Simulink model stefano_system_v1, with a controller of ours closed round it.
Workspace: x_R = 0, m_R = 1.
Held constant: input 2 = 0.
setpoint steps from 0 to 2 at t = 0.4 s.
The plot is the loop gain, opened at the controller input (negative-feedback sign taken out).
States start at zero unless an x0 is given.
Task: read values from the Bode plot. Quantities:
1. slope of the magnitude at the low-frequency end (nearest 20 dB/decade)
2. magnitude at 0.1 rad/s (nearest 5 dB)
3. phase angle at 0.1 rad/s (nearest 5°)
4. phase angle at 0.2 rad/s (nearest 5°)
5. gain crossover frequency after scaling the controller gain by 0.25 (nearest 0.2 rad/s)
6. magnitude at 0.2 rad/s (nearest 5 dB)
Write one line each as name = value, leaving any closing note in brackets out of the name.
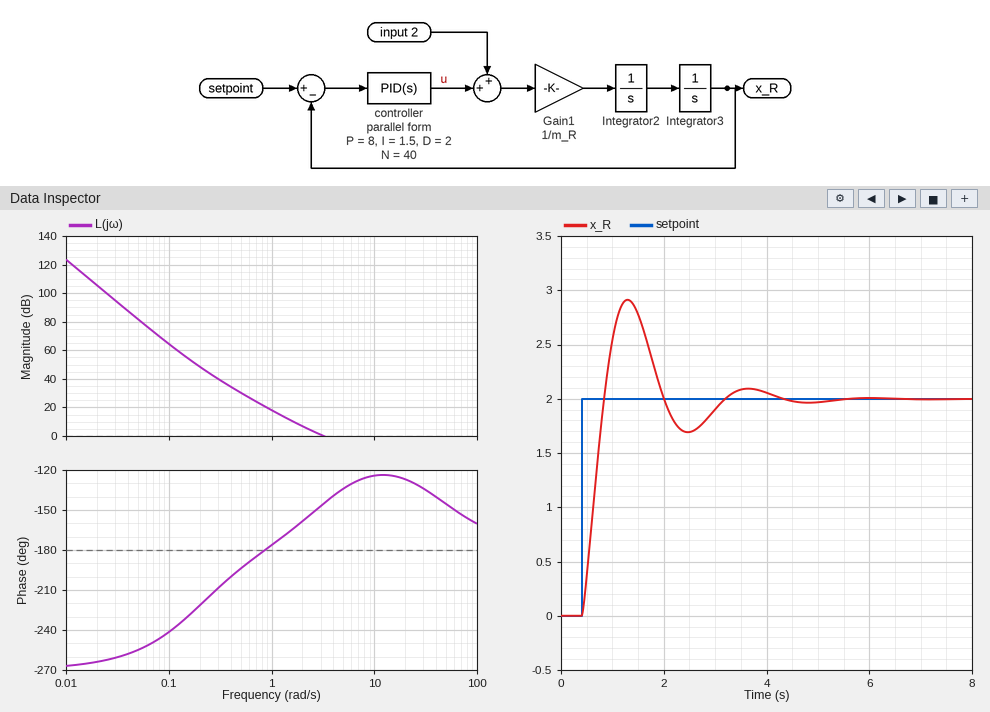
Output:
slope of the magnitude at the low-frequency end = -60 dB/decade
magnitude at 0.1 rad/s = 65 dB
phase angle at 0.1 rad/s = -240°
phase angle at 0.2 rad/s = -220°
gain crossover frequency after scaling the controller gain by 0.25 = 1.4 rad/s
magnitude at 0.2 rad/s = 50 dB
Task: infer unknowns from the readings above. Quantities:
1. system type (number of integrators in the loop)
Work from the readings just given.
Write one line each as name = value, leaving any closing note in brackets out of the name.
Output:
system type = 3
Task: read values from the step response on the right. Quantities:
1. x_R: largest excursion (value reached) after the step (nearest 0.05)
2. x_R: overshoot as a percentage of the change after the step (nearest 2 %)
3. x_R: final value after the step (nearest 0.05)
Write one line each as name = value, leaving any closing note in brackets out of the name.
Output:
x_R: largest excursion (value reached) after the step = 2.90
x_R: overshoot as a percentage of the change after the step = 46 %
x_R: final value after the step = 2.00
